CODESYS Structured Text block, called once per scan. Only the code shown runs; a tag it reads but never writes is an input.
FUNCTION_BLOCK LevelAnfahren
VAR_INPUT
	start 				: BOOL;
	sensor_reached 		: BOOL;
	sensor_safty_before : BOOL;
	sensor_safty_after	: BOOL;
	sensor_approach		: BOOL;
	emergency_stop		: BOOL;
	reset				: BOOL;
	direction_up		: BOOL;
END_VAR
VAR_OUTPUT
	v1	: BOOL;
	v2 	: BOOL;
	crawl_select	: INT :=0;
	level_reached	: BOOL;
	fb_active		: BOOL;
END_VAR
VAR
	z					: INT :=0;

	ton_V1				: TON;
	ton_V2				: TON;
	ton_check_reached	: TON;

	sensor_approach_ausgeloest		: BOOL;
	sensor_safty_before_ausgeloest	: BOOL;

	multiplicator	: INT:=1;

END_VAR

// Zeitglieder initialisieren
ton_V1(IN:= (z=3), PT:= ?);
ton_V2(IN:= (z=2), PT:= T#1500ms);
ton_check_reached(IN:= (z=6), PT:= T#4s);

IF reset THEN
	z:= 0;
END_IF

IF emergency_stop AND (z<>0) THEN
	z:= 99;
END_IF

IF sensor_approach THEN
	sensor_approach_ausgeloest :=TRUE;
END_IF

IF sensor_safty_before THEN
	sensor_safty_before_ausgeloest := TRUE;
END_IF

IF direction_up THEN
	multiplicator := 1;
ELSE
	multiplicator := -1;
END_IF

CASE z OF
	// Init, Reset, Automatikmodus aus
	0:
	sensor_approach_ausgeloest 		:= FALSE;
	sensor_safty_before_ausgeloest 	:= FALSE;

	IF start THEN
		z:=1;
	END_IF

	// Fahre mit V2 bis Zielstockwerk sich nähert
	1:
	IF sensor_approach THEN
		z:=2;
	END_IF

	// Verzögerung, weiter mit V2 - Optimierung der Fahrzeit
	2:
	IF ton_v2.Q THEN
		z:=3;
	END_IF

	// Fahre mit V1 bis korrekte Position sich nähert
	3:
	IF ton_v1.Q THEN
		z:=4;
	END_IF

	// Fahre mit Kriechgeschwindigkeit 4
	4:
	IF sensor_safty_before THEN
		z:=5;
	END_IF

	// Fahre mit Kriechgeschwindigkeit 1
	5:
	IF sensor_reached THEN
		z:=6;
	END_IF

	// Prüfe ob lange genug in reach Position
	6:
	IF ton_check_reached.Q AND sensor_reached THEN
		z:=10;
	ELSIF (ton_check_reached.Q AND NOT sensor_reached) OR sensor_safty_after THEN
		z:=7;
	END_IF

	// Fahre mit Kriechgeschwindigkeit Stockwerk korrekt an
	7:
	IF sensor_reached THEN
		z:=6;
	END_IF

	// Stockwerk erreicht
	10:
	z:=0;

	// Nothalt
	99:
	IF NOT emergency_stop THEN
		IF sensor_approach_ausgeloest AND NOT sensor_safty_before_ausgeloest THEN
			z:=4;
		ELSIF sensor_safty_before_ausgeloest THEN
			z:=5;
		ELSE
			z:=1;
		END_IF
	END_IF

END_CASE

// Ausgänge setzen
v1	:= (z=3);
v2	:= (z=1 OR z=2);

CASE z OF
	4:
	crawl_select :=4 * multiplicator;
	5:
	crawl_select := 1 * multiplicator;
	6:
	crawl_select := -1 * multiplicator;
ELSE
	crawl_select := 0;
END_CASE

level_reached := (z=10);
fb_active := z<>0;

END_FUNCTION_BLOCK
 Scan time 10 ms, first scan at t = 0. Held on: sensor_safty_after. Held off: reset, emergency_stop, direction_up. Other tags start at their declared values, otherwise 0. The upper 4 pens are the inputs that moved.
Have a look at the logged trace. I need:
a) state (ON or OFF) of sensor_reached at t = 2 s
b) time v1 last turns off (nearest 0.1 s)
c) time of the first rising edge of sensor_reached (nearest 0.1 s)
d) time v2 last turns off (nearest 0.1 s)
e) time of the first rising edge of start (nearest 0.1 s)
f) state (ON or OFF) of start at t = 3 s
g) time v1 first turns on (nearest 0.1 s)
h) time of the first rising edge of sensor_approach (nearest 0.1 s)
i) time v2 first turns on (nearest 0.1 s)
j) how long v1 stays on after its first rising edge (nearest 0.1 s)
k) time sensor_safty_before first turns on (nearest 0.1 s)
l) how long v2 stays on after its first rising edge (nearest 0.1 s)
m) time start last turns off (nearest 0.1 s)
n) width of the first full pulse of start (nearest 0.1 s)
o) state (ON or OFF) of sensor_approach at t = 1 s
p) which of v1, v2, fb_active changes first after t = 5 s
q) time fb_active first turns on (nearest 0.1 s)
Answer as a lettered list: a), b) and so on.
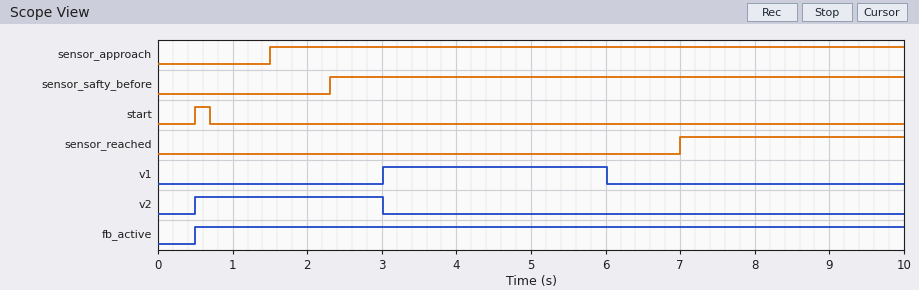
a) OFF
b) 6.0 s
c) 7.0 s
d) 3.0 s
e) 0.5 s
f) OFF
g) 3.0 s
h) 1.5 s
i) 0.5 s
j) 3.0 s
k) 2.3 s
l) 2.5 s
m) 0.7 s
n) 0.2 s
o) OFF
p) v1
q) 0.5 s
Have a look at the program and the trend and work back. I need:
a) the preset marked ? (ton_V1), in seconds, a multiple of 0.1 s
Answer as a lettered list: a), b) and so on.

a) 3.0 s
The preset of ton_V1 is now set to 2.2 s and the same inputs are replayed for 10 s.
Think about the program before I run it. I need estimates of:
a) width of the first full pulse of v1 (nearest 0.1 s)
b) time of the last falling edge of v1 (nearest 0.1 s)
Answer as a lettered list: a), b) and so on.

a) 2.2 s
b) 5.2 s
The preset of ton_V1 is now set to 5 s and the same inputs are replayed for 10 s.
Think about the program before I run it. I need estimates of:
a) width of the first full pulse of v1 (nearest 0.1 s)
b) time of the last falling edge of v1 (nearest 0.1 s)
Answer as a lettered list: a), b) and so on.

a) 5.0 s
b) 8.0 s
